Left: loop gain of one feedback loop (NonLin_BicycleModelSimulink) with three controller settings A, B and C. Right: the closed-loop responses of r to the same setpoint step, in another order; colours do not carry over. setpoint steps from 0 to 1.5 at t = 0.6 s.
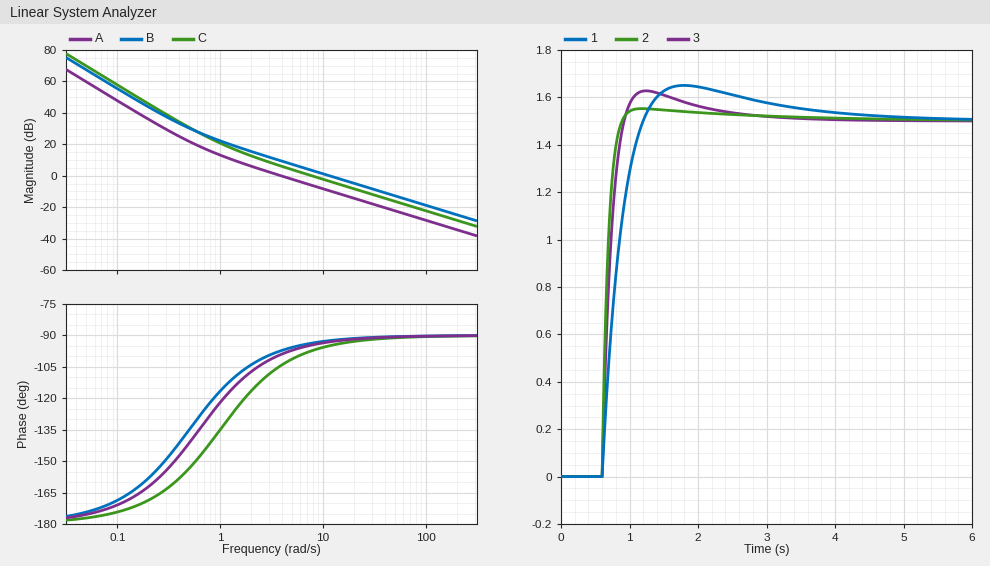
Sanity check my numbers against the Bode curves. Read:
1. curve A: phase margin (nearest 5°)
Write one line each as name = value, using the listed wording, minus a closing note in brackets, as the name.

curve A: phase margin = 80°
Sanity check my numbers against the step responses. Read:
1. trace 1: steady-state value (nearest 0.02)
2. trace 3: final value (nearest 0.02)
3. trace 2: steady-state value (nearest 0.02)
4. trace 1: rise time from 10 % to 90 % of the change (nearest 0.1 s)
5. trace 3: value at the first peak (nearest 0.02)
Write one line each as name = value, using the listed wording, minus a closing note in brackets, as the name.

trace 1: steady-state value = 1.50
trace 3: final value = 1.50
trace 2: steady-state value = 1.50
trace 1: rise time from 10 % to 90 % of the change = 0.4 s
trace 3: value at the first peak = 1.62
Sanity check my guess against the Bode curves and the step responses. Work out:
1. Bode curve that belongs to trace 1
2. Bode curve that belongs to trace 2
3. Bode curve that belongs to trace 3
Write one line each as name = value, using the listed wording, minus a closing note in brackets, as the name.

Bode curve that belongs to trace 1 = A
Bode curve that belongs to trace 2 = B
Bode curve that belongs to trace 3 = C
